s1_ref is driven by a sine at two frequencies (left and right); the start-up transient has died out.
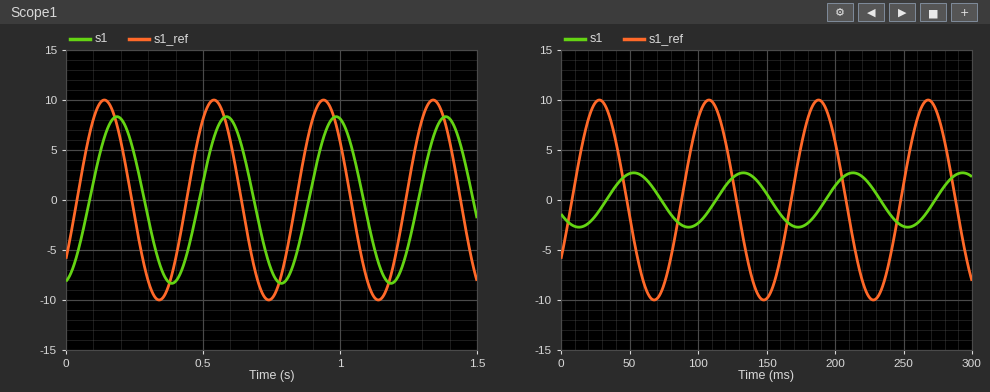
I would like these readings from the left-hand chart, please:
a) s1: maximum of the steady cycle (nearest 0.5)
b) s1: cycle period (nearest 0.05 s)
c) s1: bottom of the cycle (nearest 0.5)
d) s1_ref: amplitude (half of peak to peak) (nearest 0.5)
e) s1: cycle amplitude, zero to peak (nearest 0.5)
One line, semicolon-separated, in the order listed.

8.5; 0.40 s; -8.5; 10.0; 8.5
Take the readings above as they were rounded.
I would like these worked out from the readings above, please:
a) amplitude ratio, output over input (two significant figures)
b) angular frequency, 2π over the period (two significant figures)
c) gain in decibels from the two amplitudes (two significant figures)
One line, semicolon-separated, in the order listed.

0.85; 16 rad/s; -1.4 dB
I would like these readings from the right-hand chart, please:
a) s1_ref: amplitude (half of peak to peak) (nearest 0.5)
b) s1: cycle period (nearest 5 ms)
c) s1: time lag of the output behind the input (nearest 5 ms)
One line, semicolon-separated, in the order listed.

10.0; 80 ms; 25 ms
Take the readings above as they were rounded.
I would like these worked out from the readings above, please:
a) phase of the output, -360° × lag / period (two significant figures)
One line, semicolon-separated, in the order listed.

-110°
